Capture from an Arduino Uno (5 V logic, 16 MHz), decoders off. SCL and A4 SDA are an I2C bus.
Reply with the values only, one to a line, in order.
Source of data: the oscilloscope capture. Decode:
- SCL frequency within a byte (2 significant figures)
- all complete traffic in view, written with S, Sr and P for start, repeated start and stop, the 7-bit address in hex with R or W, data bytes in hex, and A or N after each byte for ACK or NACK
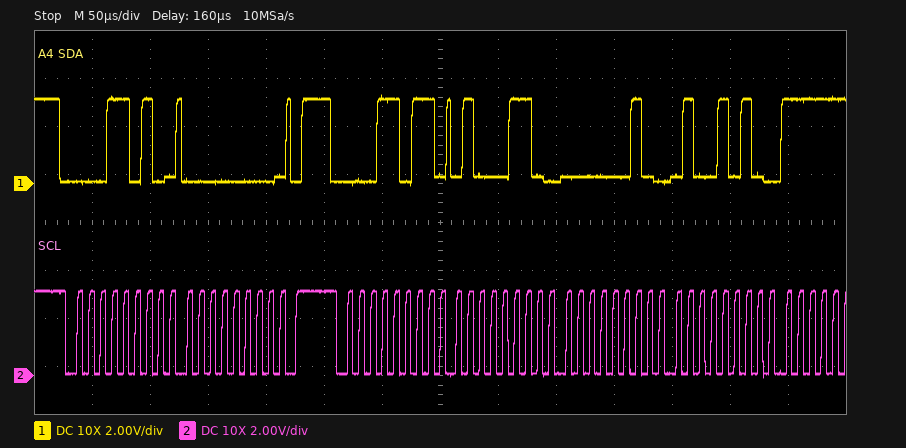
100 kHz
S 0DW A 00 A P S 0DR A 46 A 02 A 4A A
